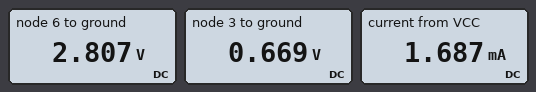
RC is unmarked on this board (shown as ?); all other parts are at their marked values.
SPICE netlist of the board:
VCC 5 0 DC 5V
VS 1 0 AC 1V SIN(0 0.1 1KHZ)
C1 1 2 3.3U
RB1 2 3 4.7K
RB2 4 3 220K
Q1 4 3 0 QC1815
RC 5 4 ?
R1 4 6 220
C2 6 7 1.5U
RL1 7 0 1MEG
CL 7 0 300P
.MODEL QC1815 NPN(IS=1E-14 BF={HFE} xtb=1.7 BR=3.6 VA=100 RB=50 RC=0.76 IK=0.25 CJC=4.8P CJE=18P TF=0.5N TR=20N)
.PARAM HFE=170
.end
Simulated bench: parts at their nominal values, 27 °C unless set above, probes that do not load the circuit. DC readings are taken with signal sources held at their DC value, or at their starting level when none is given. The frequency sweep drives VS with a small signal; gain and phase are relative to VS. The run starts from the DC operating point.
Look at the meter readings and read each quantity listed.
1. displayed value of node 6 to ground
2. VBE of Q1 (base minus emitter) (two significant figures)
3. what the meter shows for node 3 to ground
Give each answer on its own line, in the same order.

2.807 V
670 mV
0.669 V
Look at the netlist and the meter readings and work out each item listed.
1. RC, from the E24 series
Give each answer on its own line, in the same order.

1.3 kΩ
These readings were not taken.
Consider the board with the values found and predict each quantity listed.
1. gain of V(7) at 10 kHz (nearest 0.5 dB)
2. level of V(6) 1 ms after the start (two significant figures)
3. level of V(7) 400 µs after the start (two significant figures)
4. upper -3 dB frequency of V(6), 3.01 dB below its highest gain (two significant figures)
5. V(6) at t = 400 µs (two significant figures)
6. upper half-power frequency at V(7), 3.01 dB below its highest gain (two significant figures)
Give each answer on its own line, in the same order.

25.0 dB
2.8 V
-1.1 V
290 kHz
1.7 V
290 kHz
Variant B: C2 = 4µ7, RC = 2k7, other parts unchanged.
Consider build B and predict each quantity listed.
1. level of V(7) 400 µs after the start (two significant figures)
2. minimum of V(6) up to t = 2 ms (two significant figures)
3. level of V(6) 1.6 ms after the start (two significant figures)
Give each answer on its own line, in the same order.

-1.4 V
120 mV
3.4 V
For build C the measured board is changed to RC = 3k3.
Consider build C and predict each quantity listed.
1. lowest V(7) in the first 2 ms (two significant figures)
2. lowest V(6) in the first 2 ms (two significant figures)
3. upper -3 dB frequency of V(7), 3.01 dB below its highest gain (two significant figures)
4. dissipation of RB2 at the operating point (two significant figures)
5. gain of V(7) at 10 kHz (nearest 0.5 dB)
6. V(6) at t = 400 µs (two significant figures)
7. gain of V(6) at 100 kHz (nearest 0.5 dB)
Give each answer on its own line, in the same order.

-1.8 V
110 mV
180 kHz
6.7 µW
28.0 dB
330 mV
27.0 dB
